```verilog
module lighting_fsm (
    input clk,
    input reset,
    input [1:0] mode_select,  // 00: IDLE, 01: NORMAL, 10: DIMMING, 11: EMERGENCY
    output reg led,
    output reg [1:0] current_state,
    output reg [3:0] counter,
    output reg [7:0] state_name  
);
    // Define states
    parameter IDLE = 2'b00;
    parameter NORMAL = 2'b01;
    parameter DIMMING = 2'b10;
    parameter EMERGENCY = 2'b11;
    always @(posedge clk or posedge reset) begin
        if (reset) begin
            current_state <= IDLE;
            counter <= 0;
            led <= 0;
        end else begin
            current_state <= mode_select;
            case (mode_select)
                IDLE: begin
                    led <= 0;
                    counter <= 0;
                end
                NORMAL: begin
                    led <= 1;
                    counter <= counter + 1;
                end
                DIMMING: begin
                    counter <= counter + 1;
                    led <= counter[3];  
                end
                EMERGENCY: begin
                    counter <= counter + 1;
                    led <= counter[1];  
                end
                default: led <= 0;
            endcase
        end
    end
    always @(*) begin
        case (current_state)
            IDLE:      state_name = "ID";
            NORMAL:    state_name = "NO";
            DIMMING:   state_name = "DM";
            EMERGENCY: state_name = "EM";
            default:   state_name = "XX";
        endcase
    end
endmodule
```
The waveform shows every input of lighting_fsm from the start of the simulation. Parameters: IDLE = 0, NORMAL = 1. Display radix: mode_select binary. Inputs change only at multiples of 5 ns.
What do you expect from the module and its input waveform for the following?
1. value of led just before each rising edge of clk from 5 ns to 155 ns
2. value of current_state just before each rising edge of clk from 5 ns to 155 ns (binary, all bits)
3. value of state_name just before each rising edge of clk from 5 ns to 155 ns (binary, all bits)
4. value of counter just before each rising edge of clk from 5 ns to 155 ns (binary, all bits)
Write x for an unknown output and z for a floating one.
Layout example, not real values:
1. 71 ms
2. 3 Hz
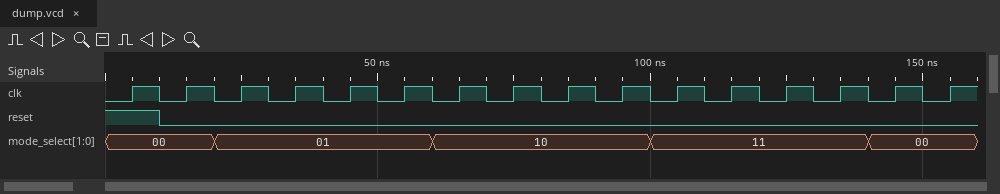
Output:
1. 0 0 0 1 1 1 1 0 0 0 0 0 0 1 1 0
2. 00, 00, 00, 01, 01, 01, 01, 10, 10, 10, 10, 11, 11, 11, 11, 00
3. 01000100, 01000100, 01000100, 01001111, 01001111, 01001111, 01001111, 01001101, 01001101, 01001101, 01001101, 01001101, 01001101, 01001101, 01001101, 01000100
4. 0000, 0000, 0000, 0001, 0010, 0011, 0100, 0101, 0110, 0111, 1000, 1001, 1010, 1011, 1100, 0000
